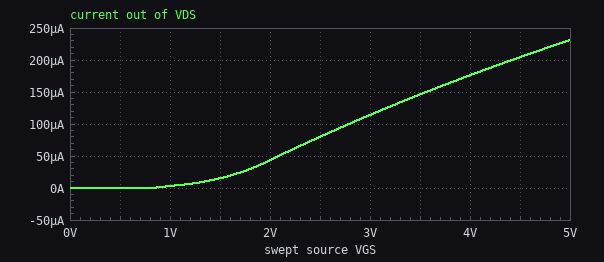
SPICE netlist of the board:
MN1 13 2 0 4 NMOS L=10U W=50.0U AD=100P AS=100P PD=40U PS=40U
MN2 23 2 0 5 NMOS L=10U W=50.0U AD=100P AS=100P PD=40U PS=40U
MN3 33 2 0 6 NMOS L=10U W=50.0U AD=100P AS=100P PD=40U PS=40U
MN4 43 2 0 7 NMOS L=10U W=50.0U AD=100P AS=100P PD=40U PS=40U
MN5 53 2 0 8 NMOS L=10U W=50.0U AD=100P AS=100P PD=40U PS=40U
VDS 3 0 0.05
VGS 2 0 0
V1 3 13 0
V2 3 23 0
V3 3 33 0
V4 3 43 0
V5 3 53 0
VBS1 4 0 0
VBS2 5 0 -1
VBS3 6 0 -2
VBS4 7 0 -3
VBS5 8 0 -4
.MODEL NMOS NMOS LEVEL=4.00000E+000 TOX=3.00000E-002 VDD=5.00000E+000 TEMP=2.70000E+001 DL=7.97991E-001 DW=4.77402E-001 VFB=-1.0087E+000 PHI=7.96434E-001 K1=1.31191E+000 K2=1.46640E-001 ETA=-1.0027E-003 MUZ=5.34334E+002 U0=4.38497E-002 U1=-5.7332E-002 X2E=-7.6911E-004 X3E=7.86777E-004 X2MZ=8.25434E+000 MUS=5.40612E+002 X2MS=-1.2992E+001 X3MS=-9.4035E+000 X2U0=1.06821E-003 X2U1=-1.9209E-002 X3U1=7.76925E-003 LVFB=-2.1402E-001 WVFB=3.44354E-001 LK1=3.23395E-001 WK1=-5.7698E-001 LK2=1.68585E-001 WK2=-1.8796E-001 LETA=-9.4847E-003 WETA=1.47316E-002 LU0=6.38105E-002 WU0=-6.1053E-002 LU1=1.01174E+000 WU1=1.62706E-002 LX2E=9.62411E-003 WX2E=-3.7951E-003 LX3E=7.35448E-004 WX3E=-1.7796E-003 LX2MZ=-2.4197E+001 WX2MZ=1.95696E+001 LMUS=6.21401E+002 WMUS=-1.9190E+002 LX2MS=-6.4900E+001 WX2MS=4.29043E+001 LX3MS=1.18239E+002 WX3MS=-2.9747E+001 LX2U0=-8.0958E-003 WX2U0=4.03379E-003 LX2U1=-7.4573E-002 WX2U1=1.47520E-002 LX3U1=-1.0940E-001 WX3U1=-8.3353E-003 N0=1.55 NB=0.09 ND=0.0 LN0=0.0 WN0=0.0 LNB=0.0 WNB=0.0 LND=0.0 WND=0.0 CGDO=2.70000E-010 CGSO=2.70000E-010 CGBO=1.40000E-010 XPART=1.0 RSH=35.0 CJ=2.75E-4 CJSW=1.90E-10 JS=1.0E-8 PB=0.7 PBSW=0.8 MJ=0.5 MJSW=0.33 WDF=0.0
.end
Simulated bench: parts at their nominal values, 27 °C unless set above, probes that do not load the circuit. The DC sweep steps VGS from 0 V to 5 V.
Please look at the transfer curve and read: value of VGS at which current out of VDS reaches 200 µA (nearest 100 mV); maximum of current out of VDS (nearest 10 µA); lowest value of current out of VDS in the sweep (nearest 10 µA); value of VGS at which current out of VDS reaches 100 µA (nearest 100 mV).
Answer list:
4.4 V
230 µA
0 A
2.8 V
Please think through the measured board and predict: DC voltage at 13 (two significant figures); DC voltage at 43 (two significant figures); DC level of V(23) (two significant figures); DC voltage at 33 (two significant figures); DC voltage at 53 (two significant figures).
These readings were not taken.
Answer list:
50 mV
50 mV
50 mV
50 mV
50 mV
